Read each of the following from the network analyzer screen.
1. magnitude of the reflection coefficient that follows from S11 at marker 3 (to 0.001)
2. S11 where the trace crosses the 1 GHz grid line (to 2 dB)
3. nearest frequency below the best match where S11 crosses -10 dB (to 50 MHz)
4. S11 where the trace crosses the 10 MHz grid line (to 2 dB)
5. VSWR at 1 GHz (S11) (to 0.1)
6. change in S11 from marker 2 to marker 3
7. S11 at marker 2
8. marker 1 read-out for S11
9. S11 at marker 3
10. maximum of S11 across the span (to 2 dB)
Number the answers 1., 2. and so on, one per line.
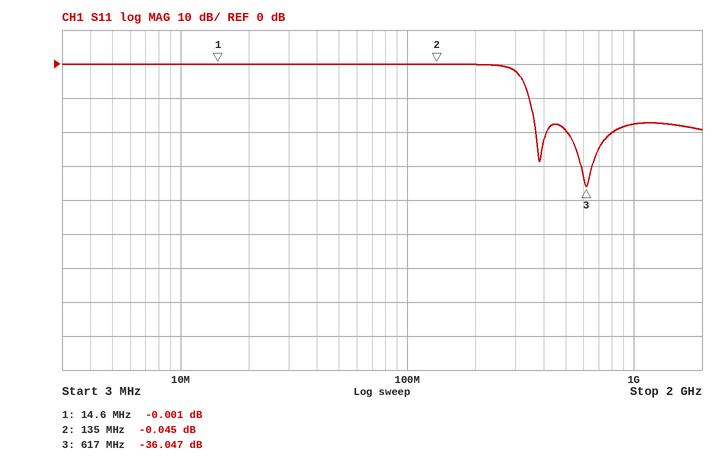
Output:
1. 0.016
2. -18 dB
3. 350 MHz
4. 0 dB
5. 1.3
6. -36.002 dB
7. -0.045 dB
8. -0.001 dB
9. -36.047 dB
10. 0 dB
